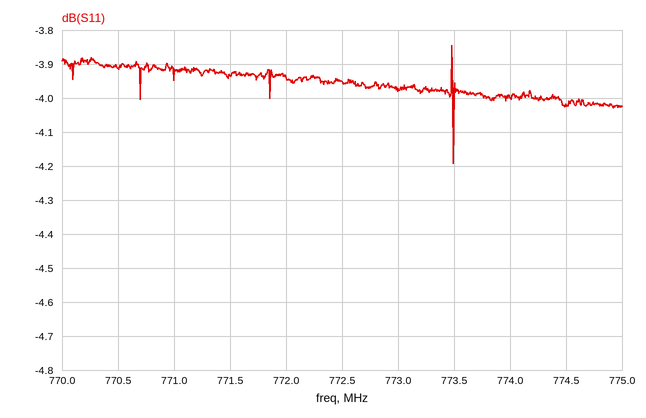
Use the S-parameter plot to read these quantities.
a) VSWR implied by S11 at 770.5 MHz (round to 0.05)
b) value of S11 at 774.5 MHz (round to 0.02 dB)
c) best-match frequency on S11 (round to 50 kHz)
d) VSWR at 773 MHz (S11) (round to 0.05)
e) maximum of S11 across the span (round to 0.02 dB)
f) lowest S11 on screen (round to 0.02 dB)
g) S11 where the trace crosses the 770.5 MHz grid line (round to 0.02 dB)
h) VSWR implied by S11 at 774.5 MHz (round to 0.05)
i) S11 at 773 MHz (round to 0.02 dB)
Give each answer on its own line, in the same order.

4.50
-4.02 dB
773.50 MHz
4.45
-3.84 dB
-4.20 dB
-3.92 dB
4.40
-3.98 dB
